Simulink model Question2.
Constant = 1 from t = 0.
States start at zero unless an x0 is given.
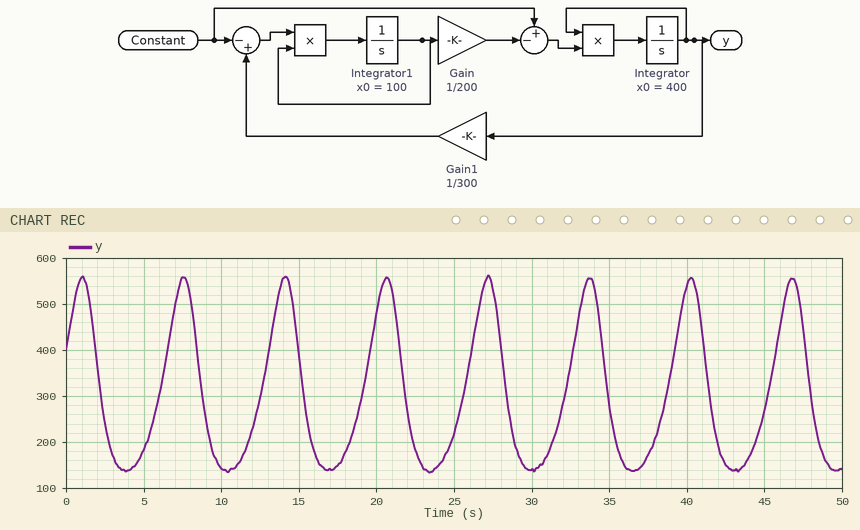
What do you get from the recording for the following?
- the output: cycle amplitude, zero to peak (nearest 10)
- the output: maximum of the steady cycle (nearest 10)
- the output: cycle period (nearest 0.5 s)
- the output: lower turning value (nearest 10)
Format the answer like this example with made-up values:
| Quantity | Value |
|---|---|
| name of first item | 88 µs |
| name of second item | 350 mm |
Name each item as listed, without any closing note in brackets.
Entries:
| Quantity | Value |
|---|---|
| the output: cycle amplitude, zero to peak | 210 |
| the output: maximum of the steady cycle | 560 |
| the output: cycle period | 6.5 s |
| the output: lower turning value | 140 |
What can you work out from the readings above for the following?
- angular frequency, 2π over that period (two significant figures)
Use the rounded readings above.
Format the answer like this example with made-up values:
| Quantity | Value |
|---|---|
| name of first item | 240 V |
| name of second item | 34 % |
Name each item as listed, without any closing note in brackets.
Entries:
| Quantity | Value |
|---|---|
| angular frequency, 2π over that period | 0.97 rad/s |
